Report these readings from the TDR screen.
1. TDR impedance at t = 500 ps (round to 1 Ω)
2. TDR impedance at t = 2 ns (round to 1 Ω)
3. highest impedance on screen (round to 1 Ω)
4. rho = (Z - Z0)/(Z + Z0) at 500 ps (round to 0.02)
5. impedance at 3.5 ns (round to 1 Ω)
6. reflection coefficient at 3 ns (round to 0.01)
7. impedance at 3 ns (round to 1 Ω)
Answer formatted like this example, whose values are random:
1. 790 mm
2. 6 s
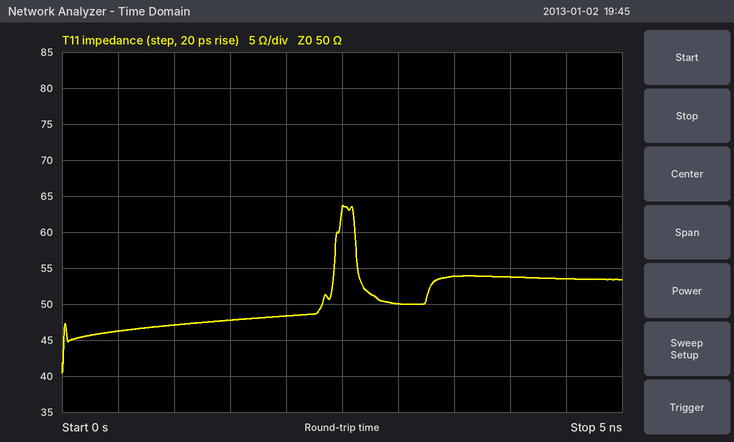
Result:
1. 46 Ω
2. 48 Ω
3. 64 Ω
4. -0.04
5. 54 Ω
6. 0.00
7. 50 Ω
